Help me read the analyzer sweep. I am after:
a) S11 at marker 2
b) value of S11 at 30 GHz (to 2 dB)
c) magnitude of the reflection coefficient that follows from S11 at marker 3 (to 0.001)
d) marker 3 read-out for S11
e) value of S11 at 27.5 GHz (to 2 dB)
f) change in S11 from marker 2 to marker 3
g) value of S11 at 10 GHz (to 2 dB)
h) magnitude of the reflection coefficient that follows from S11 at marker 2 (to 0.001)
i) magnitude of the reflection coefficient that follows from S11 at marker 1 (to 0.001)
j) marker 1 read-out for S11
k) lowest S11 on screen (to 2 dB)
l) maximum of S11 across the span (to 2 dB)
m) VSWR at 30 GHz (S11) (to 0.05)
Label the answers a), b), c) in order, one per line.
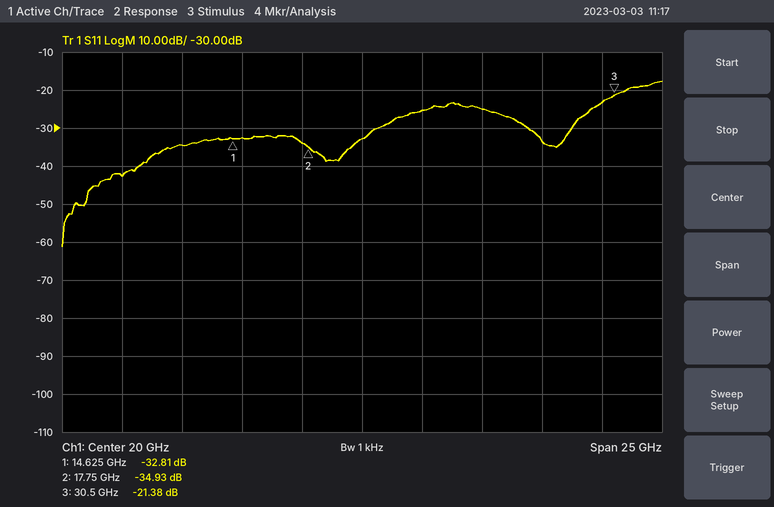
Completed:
a) -34.93 dB
b) -24 dB
c) 0.085
d) -21.38 dB
e) -34 dB
f) 13.55 dB
g) -42 dB
h) 0.018
i) 0.023
j) -32.81 dB
k) -62 dB
l) -18 dB
m) 1.15
